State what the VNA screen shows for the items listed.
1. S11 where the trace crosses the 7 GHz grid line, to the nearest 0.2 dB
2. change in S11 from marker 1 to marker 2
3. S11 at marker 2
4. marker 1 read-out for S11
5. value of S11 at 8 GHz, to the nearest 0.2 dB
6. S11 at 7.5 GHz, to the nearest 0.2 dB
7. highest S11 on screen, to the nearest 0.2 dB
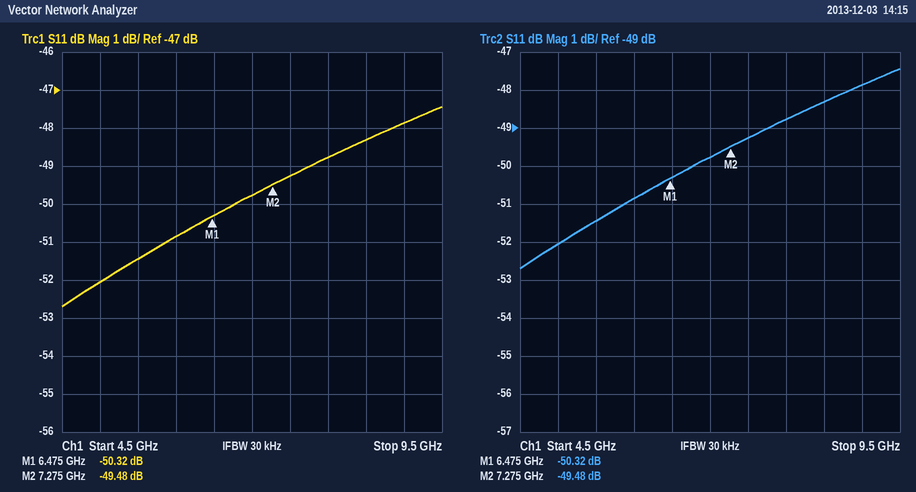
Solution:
-49.8 dB
0.84 dB
-49.48 dB
-50.32 dB
-48.8 dB
-49.2 dB
-47.4 dB
